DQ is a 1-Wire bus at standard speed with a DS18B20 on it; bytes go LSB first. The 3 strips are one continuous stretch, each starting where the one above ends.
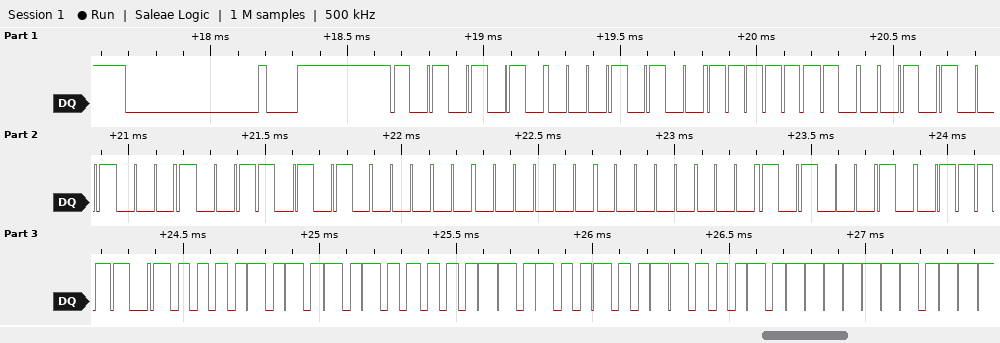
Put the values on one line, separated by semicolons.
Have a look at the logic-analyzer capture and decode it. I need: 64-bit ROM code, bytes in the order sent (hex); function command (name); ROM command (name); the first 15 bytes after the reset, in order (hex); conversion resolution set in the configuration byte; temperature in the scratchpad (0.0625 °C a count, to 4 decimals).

28 7F 94 C8 0A 00 00 45; Read Scratchpad; Match ROM; 55 28 7F 94 C8 0A 00 00 45 BE 50 05 4B 46 7F; 12 bits; 85.0000 °C
